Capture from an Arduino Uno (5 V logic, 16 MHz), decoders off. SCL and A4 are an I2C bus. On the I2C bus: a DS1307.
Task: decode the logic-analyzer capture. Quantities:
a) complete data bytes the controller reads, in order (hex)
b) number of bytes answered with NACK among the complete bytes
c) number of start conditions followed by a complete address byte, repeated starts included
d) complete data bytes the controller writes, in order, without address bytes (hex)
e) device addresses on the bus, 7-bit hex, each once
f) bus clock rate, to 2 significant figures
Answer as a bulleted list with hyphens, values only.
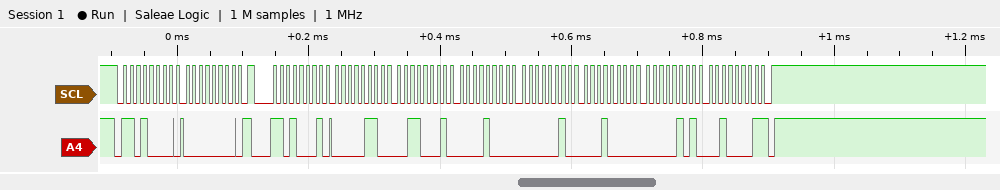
- 06 31 08 02 10 05 21
- 1
- 2
- 00
- 0x68
- 100 kHz
